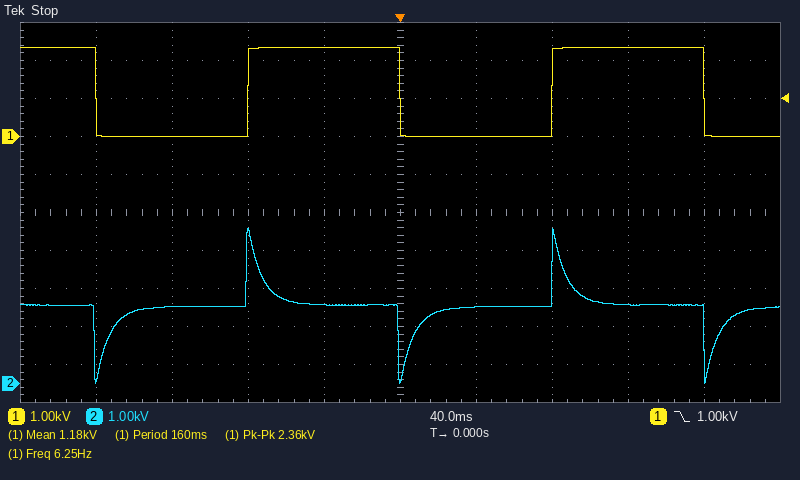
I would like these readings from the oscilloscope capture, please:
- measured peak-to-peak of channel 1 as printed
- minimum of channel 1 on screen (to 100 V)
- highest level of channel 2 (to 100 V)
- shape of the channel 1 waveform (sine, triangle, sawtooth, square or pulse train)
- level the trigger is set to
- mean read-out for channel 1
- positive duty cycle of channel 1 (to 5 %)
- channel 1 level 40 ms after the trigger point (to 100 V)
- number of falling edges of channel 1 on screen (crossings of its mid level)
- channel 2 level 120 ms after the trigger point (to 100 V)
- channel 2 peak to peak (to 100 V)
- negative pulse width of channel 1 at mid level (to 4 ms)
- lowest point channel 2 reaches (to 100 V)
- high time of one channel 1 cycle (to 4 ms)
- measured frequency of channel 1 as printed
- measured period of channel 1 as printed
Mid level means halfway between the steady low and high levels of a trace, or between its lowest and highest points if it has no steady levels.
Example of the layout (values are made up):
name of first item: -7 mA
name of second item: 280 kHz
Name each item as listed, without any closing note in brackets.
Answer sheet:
measured peak-to-peak of channel 1 as printed: 2.36 kV
minimum of channel 1 on screen: 0.0 kV
highest level of channel 2: 4.1 kV
shape of the channel 1 waveform: square
level the trigger is set to: 1.00 kV
mean read-out for channel 1: 1.18 kV
positive duty cycle of channel 1: 50 %
channel 1 level 40 ms after the trigger point: 0.0 kV
number of falling edges of channel 1 on screen: 3
channel 2 level 120 ms after the trigger point: 2.1 kV
channel 2 peak to peak: 4.1 kV
negative pulse width of channel 1 at mid level: 80 ms
lowest point channel 2 reaches: 0.0 kV
high time of one channel 1 cycle: 80 ms
measured frequency of channel 1 as printed: 6.25 Hz
measured period of channel 1 as printed: 160 ms
